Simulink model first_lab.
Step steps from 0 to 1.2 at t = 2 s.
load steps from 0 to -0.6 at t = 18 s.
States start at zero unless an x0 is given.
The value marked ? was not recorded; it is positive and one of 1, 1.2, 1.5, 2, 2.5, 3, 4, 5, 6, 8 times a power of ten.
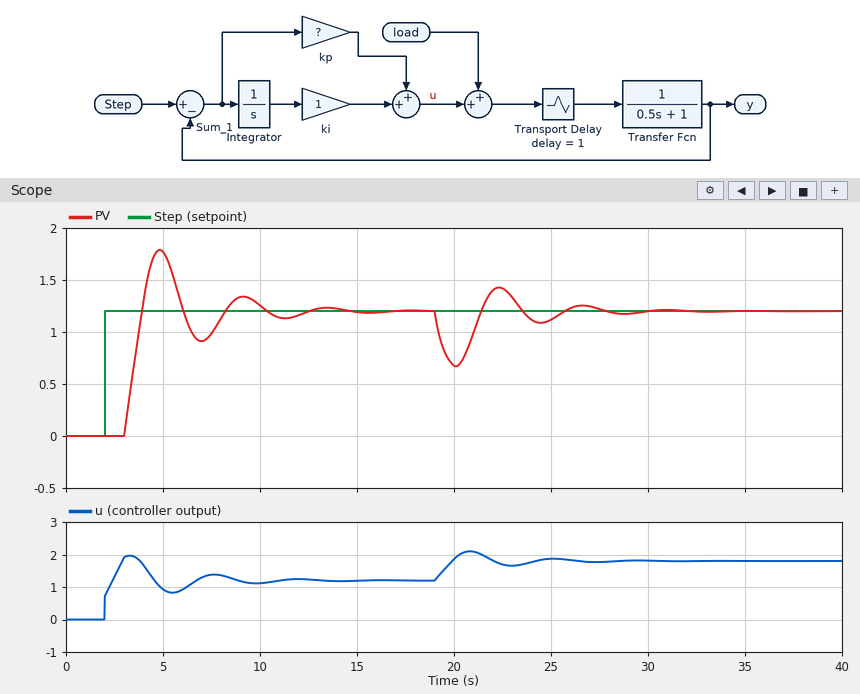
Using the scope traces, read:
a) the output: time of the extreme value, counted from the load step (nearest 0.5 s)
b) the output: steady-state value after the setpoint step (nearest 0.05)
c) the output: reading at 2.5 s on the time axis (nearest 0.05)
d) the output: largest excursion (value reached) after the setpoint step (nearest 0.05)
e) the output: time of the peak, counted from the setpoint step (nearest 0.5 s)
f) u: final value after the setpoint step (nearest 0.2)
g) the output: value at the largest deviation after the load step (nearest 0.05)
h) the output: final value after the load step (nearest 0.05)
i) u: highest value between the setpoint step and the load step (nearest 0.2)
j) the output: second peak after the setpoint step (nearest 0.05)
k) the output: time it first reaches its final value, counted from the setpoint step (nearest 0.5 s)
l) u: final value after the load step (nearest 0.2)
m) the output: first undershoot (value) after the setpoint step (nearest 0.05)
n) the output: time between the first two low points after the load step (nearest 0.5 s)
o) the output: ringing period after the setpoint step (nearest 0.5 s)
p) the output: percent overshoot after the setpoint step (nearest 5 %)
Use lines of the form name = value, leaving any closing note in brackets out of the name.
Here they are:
the output: time of the extreme value, counted from the load step = 2.0 s
the output: steady-state value after the setpoint step = 1.20
the output: reading at 2.5 s on the time axis = 0.00
the output: largest excursion (value reached) after the setpoint step = 1.80
the output: time of the peak, counted from the setpoint step = 3.0 s
u: final value after the setpoint step = 1.2
the output: value at the largest deviation after the load step = 0.65
the output: final value after the load step = 1.20
u: highest value between the setpoint step and the load step = 2.0
the output: second peak after the setpoint step = 1.35
the output: time it first reaches its final value, counted from the setpoint step = 2.0 s
u: final value after the load step = 1.8
the output: first undershoot (value) after the setpoint step = 0.90
the output: time between the first two low points after the load step = 4.5 s
the output: ringing period after the setpoint step = 4.5 s
the output: percent overshoot after the setpoint step = 50 %
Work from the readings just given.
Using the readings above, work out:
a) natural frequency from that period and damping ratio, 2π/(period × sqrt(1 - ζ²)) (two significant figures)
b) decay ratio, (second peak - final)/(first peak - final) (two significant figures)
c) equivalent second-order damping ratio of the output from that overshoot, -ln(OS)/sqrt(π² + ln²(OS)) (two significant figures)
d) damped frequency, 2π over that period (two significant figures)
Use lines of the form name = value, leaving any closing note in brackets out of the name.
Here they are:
natural frequency from that period and damping ratio, 2π/(period × sqrt(1 - ζ²)) = 1.4 rad/s
decay ratio, (second peak - final)/(first peak - final) = 0.25
equivalent second-order damping ratio of the output from that overshoot, -ln(OS)/sqrt(π² + ln²(OS)) = 0.22
damped frequency, 2π over that period = 1.4 rad/s
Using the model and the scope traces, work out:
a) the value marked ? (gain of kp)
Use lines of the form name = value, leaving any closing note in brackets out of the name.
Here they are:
the value marked ? = 0.6
